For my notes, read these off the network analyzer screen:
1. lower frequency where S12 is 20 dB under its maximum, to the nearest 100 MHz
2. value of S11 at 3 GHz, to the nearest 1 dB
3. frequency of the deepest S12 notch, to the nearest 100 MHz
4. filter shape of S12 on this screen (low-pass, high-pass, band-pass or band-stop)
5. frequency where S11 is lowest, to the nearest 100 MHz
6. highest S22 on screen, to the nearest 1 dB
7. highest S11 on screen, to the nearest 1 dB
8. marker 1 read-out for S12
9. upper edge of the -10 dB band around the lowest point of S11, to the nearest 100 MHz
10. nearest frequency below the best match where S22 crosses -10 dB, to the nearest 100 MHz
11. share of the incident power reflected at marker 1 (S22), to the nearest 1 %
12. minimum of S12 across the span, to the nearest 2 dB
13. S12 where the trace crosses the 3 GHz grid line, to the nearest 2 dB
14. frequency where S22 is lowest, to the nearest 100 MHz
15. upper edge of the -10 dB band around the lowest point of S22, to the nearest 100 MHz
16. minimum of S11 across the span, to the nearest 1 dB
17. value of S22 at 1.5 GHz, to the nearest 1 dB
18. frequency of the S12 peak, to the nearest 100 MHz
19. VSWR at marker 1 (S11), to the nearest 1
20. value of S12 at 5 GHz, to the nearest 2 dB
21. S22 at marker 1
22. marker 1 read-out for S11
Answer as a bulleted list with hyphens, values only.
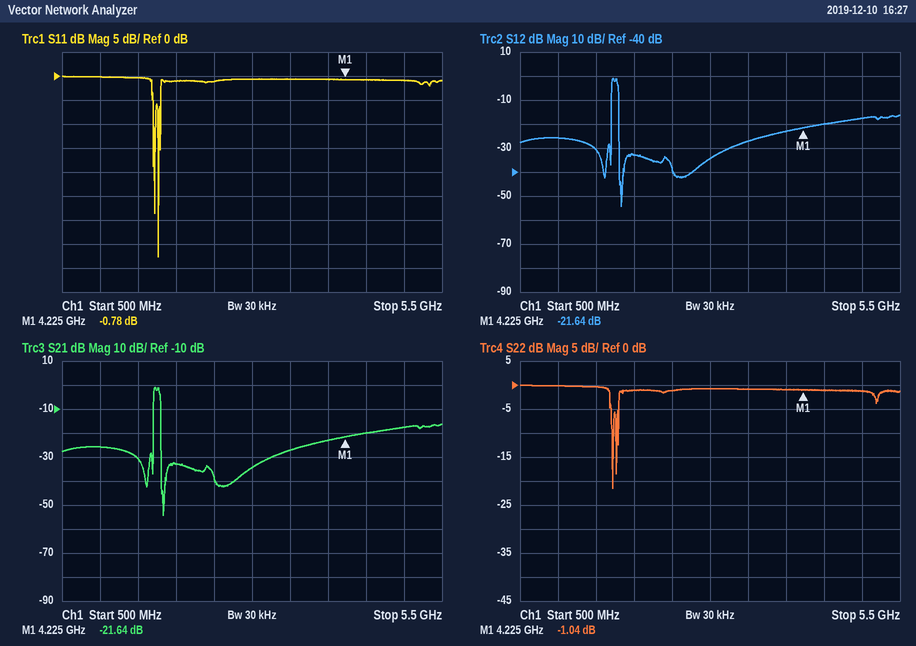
- 1.7 GHz
- -1 dB
- 1.8 GHz
- band-pass
- 1.8 GHz
- 0 dB
- 0 dB
- -21.64 dB
- 1.8 GHz
- 1.7 GHz
- 79 %
- -54 dB
- -34 dB
- 1.7 GHz
- 1.7 GHz
- -38 dB
- 0 dB
- 1.7 GHz
- 22
- -18 dB
- -1.04 dB
- -0.78 dB
